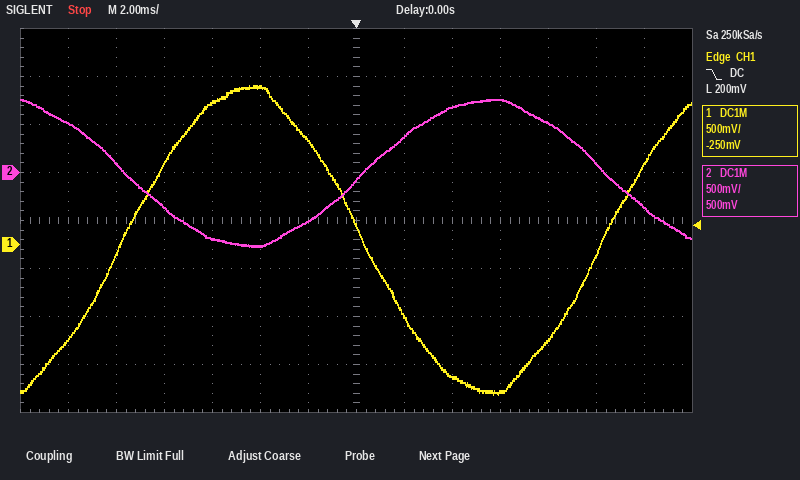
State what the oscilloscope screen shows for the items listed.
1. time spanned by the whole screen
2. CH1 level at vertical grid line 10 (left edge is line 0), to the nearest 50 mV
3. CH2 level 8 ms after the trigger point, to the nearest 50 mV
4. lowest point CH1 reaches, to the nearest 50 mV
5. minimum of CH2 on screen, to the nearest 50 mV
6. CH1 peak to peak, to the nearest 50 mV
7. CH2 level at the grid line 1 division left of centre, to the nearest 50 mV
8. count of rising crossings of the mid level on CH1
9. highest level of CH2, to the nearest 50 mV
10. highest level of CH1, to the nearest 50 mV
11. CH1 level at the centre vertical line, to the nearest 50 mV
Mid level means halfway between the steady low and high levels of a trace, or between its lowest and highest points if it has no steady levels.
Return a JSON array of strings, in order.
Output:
["28 ms", "-1.55 V", "500 mV", "-1.55 V", "-750 mV", "3.20 V", "-500 mV", "2", "750 mV", "1.65 V", "200 mV"]
